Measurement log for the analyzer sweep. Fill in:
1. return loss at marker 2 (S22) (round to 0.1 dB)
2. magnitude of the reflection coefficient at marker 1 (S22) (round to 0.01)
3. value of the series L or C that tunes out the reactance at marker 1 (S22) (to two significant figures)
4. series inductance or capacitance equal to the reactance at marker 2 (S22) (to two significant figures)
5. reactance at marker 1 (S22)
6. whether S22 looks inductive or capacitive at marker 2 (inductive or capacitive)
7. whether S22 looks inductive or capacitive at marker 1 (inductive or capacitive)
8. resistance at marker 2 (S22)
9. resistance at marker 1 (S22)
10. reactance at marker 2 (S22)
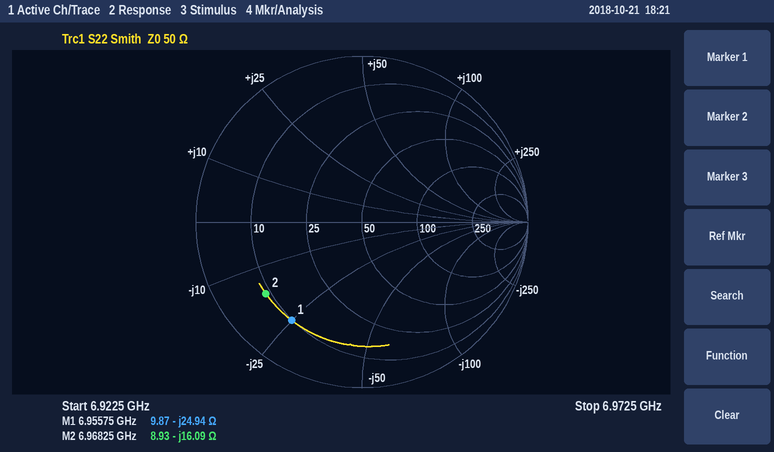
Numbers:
2.8 dB
0.73
570 pH
1.4 pF
-24.94 Ω
capacitive
capacitive
8.93 Ω
9.87 Ω
-16.09 Ω
